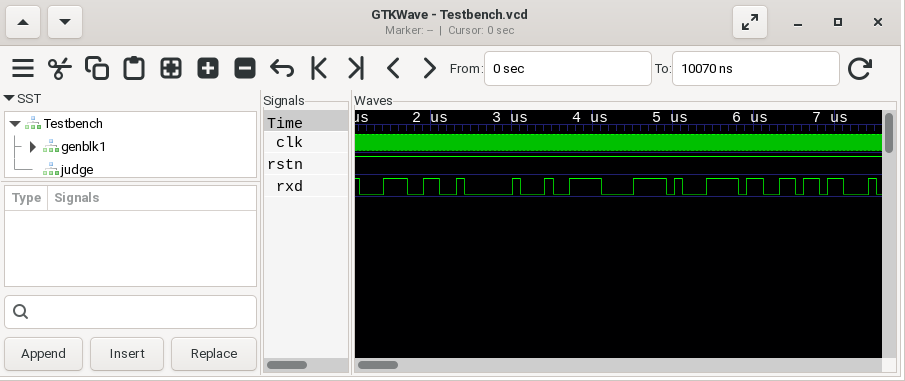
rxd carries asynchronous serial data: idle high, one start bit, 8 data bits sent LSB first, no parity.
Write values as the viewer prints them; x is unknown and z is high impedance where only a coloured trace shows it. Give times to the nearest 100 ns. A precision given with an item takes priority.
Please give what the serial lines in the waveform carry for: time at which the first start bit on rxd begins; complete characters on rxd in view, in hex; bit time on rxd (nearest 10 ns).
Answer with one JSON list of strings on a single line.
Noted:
["1100 ns", "9C, 02, E4, 78, BC, B6", "100 ns"]
